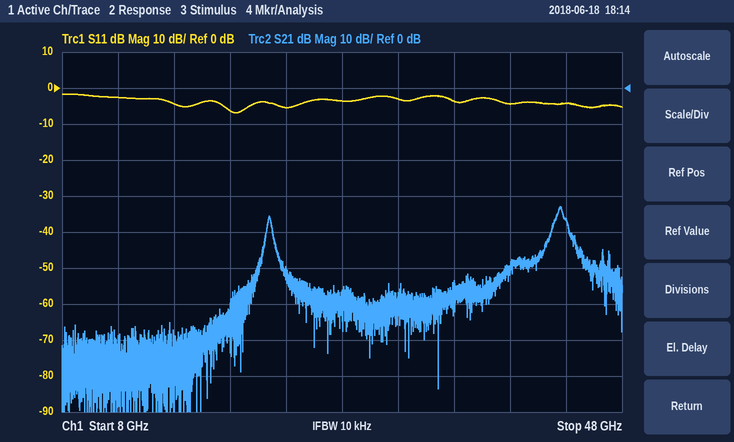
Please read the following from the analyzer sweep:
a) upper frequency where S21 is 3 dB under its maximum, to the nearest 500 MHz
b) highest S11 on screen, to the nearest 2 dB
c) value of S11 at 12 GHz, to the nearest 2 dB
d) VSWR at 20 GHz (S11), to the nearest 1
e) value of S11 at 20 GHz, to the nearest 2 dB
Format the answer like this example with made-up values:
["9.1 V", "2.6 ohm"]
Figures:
["44.0 GHz", "-2 dB", "-2 dB", "3", "-6 dB"]
